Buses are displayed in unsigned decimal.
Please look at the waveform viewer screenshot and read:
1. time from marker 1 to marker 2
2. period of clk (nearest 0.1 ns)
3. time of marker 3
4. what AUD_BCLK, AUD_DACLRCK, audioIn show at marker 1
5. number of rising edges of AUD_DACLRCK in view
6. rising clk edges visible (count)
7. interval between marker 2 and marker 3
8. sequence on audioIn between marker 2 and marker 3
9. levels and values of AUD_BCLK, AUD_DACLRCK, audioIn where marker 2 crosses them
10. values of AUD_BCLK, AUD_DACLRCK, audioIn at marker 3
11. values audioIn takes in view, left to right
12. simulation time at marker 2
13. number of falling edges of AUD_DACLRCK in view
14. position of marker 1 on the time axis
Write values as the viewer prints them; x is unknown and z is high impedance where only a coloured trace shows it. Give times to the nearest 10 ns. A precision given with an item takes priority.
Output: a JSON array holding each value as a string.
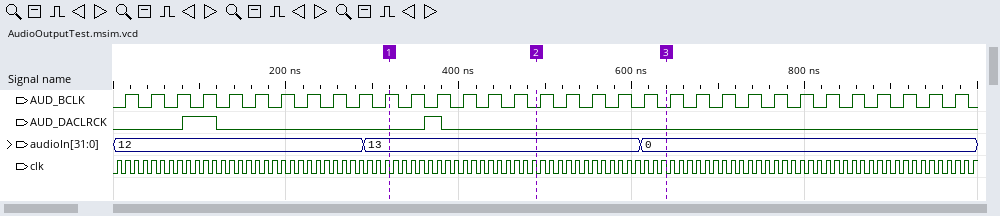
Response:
["170 ns", "10 ns", "640 ns", "AUD_BCLK=1, AUD_DACLRCK=0, audioIn=13", "2", "100", "150 ns", "13, 0", "AUD_BCLK=0, AUD_DACLRCK=0, audioIn=13", "AUD_BCLK=0, AUD_DACLRCK=0, audioIn=0", "12, 13, 0", "490 ns", "2", "320 ns"]
